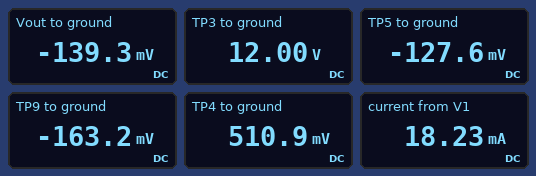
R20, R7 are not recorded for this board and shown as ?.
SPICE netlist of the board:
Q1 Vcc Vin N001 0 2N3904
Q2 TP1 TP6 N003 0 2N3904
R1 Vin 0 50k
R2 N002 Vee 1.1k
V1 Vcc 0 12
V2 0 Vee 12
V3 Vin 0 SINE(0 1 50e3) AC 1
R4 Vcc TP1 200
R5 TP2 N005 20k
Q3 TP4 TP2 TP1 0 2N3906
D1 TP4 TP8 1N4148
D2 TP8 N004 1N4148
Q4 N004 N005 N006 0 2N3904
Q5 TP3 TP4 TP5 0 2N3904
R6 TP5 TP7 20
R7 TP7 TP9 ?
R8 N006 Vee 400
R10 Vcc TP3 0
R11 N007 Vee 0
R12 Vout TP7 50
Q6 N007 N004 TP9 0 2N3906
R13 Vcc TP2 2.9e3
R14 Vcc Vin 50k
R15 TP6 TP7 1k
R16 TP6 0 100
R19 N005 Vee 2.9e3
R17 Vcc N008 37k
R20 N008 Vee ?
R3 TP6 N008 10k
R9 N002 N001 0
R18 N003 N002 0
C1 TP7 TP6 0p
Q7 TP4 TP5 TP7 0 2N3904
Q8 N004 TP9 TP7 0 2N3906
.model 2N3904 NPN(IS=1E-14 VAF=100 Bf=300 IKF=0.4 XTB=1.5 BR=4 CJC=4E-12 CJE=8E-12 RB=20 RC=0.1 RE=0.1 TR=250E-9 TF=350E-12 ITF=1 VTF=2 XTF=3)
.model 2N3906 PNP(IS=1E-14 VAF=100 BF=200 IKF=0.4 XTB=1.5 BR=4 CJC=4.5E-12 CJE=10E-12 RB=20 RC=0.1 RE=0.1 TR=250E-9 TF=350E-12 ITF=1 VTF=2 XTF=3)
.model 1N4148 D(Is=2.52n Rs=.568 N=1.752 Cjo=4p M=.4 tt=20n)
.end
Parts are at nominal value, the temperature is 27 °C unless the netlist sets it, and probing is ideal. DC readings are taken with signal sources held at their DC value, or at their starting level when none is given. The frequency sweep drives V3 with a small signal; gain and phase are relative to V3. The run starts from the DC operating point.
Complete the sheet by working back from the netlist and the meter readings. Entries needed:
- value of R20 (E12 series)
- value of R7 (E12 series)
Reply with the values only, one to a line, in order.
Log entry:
82 kΩ
33 Ω
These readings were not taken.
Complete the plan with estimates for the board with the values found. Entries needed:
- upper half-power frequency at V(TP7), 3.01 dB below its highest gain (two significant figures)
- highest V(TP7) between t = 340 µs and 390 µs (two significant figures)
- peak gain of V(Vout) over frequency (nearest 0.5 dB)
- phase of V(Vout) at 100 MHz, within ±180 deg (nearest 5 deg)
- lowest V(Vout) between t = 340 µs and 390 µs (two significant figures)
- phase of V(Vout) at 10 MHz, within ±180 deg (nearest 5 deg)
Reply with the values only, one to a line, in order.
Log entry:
28 MHz
9.9 V
21.0 dB
-110 deg
-10 V
-25 deg
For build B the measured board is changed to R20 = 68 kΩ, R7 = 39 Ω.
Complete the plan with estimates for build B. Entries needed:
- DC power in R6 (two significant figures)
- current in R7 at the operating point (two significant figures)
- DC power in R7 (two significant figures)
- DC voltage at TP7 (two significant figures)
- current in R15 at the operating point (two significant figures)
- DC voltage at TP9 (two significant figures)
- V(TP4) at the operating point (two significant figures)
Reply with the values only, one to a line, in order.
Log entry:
6.4 µW
680 µA
18 µW
-120 mV
110 µA
-140 mV
530 mV
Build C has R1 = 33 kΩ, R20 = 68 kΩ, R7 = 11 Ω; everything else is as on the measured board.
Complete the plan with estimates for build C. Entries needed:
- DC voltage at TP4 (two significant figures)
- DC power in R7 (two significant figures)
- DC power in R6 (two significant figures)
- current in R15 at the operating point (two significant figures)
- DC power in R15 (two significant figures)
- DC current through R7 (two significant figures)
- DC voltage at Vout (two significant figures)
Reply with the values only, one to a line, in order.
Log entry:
540 mV
8.2 µW
11 µW
110 µA
13 µW
860 µA
-120 mV
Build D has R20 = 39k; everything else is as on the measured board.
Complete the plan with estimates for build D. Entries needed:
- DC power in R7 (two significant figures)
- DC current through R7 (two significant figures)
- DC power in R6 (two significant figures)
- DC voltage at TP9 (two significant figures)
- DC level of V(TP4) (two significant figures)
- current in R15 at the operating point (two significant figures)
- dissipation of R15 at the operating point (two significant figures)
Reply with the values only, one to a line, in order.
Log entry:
15 µW
670 µA
8.4 µW
-45 mV
630 mV
20 µA
410 nW
